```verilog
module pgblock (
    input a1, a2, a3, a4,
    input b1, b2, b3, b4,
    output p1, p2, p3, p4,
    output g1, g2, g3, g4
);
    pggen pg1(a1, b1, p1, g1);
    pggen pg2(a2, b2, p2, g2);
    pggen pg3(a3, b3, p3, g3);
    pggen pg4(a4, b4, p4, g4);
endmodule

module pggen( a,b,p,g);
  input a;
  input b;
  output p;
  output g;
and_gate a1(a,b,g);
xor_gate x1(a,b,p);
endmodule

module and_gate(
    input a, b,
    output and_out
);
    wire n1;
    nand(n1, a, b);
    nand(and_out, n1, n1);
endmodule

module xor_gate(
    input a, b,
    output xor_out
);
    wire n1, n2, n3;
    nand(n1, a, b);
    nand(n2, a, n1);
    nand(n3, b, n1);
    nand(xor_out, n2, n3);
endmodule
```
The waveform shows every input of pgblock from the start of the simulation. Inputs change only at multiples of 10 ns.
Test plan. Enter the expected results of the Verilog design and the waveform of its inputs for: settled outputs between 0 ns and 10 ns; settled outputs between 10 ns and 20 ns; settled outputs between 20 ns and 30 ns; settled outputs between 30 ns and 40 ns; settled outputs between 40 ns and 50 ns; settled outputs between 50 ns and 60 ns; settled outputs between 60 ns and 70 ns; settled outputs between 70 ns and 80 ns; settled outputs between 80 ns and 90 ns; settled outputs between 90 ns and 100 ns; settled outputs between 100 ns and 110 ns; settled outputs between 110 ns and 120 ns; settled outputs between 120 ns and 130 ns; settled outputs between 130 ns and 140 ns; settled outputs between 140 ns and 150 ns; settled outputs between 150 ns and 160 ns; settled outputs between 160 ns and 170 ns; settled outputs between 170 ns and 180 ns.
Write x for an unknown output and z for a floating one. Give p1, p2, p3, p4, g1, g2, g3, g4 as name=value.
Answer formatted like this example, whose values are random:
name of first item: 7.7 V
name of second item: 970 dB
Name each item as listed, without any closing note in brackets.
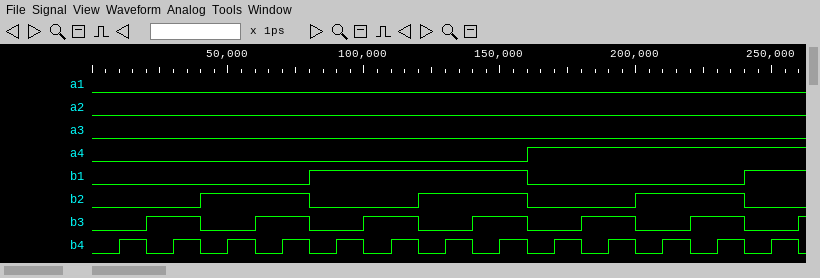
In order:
settled outputs between 0 ns and 10 ns: p1=0, p2=0, p3=0, p4=0, g1=0, g2=0, g3=0, g4=0
settled outputs between 10 ns and 20 ns: p1=0, p2=0, p3=0, p4=1, g1=0, g2=0, g3=0, g4=0
settled outputs between 20 ns and 30 ns: p1=0, p2=0, p3=1, p4=0, g1=0, g2=0, g3=0, g4=0
settled outputs between 30 ns and 40 ns: p1=0, p2=0, p3=1, p4=1, g1=0, g2=0, g3=0, g4=0
settled outputs between 40 ns and 50 ns: p1=0, p2=1, p3=0, p4=0, g1=0, g2=0, g3=0, g4=0
settled outputs between 50 ns and 60 ns: p1=0, p2=1, p3=0, p4=1, g1=0, g2=0, g3=0, g4=0
settled outputs between 60 ns and 70 ns: p1=0, p2=1, p3=1, p4=0, g1=0, g2=0, g3=0, g4=0
settled outputs between 70 ns and 80 ns: p1=0, p2=1, p3=1, p4=1, g1=0, g2=0, g3=0, g4=0
settled outputs between 80 ns and 90 ns: p1=1, p2=0, p3=0, p4=0, g1=0, g2=0, g3=0, g4=0
settled outputs between 90 ns and 100 ns: p1=1, p2=0, p3=0, p4=1, g1=0, g2=0, g3=0, g4=0
settled outputs between 100 ns and 110 ns: p1=1, p2=0, p3=1, p4=0, g1=0, g2=0, g3=0, g4=0
settled outputs between 110 ns and 120 ns: p1=1, p2=0, p3=1, p4=1, g1=0, g2=0, g3=0, g4=0
settled outputs between 120 ns and 130 ns: p1=1, p2=1, p3=0, p4=0, g1=0, g2=0, g3=0, g4=0
settled outputs between 130 ns and 140 ns: p1=1, p2=1, p3=0, p4=1, g1=0, g2=0, g3=0, g4=0
settled outputs between 140 ns and 150 ns: p1=1, p2=1, p3=1, p4=0, g1=0, g2=0, g3=0, g4=0
settled outputs between 150 ns and 160 ns: p1=1, p2=1, p3=1, p4=1, g1=0, g2=0, g3=0, g4=0
settled outputs between 160 ns and 170 ns: p1=0, p2=0, p3=0, p4=1, g1=0, g2=0, g3=0, g4=0
settled outputs between 170 ns and 180 ns: p1=0, p2=0, p3=0, p4=0, g1=0, g2=0, g3=0, g4=1
